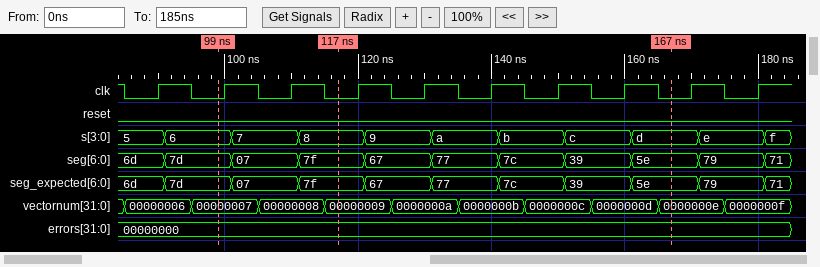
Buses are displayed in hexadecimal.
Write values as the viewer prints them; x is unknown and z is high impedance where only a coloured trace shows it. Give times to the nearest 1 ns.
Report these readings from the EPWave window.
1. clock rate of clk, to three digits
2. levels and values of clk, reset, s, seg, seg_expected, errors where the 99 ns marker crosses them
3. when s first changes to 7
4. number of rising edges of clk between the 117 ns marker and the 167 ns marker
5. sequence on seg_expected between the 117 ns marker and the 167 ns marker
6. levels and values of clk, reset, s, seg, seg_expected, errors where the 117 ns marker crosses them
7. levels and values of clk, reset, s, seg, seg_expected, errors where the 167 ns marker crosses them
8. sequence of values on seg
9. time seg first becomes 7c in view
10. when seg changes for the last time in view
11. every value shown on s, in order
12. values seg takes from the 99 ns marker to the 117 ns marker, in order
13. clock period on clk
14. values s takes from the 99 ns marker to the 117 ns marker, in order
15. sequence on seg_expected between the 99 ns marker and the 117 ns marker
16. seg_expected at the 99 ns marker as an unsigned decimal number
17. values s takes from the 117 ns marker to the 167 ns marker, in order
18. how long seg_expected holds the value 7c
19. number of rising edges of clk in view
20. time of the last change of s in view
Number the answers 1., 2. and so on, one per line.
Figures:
1. 100 MHz
2. clk=0, reset=0, s=6, seg=7d, seg_expected=7d, errors=00000000
3. 101 ns
4. 5
5. 7f, 67, 77, 7c, 39, 5e
6. clk=0, reset=0, s=8, seg=7f, seg_expected=7f, errors=00000000
7. clk=0, reset=0, s=d, seg=5e, seg_expected=5e, errors=00000000
8. 6d, 7d, 07, 7f, 67, 77, 7c, 39, 5e, 79, 71
9. 141 ns
10. 181 ns
11. 5, 6, 7, 8, 9, a, b, c, d, e, f
12. 7d, 07, 7f
13. 10 ns
14. 6, 7, 8
15. 7d, 07, 7f
16. 125
17. 8, 9, a, b, c, d
18. 10 ns
19. 10
20. 181 ns
